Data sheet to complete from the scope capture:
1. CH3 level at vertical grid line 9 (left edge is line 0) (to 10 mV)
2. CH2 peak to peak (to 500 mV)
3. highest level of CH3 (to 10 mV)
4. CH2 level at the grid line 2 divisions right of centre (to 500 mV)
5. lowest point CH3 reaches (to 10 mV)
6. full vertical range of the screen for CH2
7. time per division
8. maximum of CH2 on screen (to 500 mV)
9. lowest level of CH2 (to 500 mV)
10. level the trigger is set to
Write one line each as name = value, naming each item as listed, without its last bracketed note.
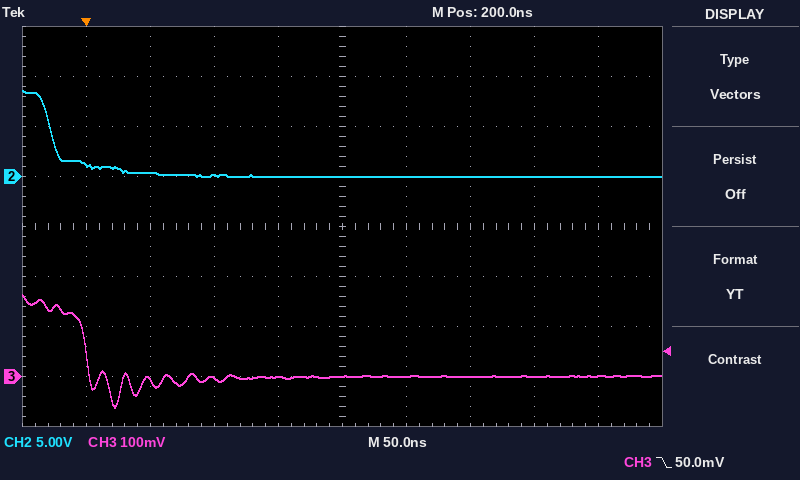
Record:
CH3 level at vertical grid line 9 (left edge is line 0) = 0 mV
CH2 peak to peak = 8.5 V
highest level of CH3 = 160 mV
CH2 level at the grid line 2 divisions right of centre = 0.0 V
lowest point CH3 reaches = -60 mV
full vertical range of the screen for CH2 = 40 V
time per division = 50 ns
maximum of CH2 on screen = 8.5 V
lowest level of CH2 = 0.0 V
level the trigger is set to = 50.0 mV
